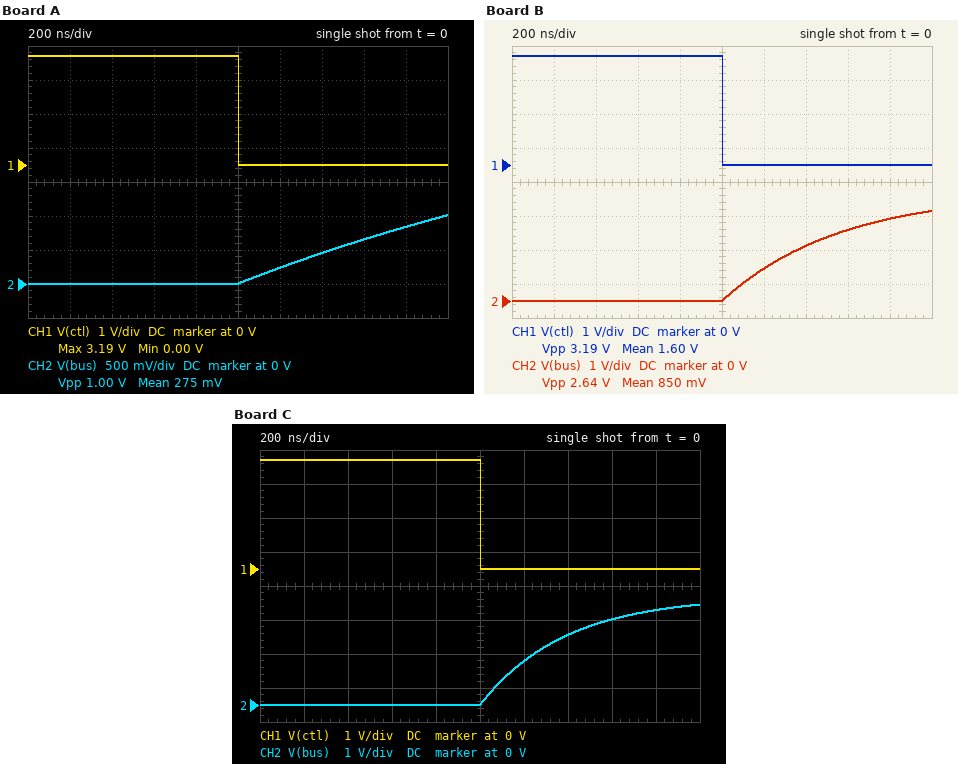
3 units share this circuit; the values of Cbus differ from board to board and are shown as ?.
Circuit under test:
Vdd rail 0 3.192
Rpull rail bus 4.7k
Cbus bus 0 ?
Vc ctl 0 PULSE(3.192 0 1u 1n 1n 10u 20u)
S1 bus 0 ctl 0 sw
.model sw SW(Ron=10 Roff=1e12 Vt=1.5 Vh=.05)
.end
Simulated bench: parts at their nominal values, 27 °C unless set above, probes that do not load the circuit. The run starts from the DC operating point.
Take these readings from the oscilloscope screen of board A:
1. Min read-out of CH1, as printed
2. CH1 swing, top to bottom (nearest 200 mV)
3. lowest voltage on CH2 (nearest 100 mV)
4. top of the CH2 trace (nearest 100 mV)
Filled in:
0.00 V
3.2 V
0 V
1.0 V
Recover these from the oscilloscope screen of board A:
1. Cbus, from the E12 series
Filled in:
560 pF
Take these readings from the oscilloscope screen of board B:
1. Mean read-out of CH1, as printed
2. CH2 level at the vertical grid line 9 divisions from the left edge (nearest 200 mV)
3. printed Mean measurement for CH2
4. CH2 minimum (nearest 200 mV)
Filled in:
1.60 V
2.4 V
850 mV
0 V
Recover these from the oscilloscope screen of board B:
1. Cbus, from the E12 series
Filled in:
120 pF
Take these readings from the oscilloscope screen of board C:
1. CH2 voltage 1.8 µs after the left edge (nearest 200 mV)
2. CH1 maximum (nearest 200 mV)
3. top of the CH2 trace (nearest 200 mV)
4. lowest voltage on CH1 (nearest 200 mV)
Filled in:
2.8 V
3.2 V
3.0 V
0 V
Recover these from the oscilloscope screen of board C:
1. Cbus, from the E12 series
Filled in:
82 pF
